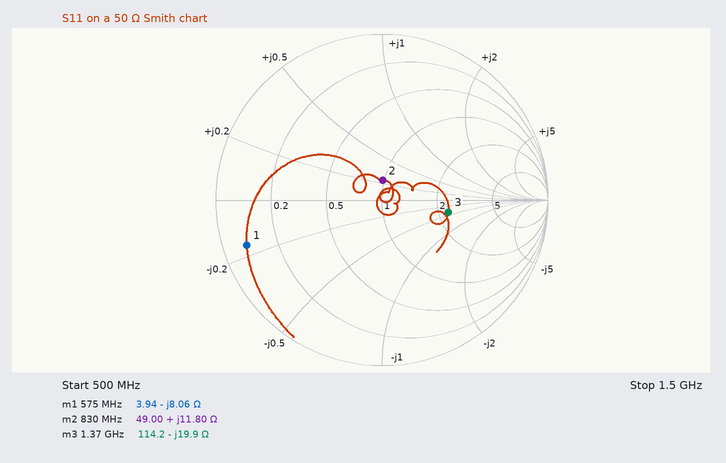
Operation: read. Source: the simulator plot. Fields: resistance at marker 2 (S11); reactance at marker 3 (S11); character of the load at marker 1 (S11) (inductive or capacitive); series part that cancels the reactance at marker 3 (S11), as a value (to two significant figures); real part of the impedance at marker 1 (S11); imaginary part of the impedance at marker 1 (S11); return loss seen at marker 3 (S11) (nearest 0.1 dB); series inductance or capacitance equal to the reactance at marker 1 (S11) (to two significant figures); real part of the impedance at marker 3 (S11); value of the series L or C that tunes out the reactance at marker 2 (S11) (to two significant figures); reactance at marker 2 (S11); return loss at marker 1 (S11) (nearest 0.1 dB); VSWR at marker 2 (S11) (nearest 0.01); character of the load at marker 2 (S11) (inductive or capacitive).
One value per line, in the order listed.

49.00 Ω
-19.9 Ω
capacitive
2.3 nH
3.94 Ω
-8.06 Ω
7.8 dB
34 pF
114.2 Ω
16 pF
+11.80 Ω
1.3 dB
1.27
inductive
